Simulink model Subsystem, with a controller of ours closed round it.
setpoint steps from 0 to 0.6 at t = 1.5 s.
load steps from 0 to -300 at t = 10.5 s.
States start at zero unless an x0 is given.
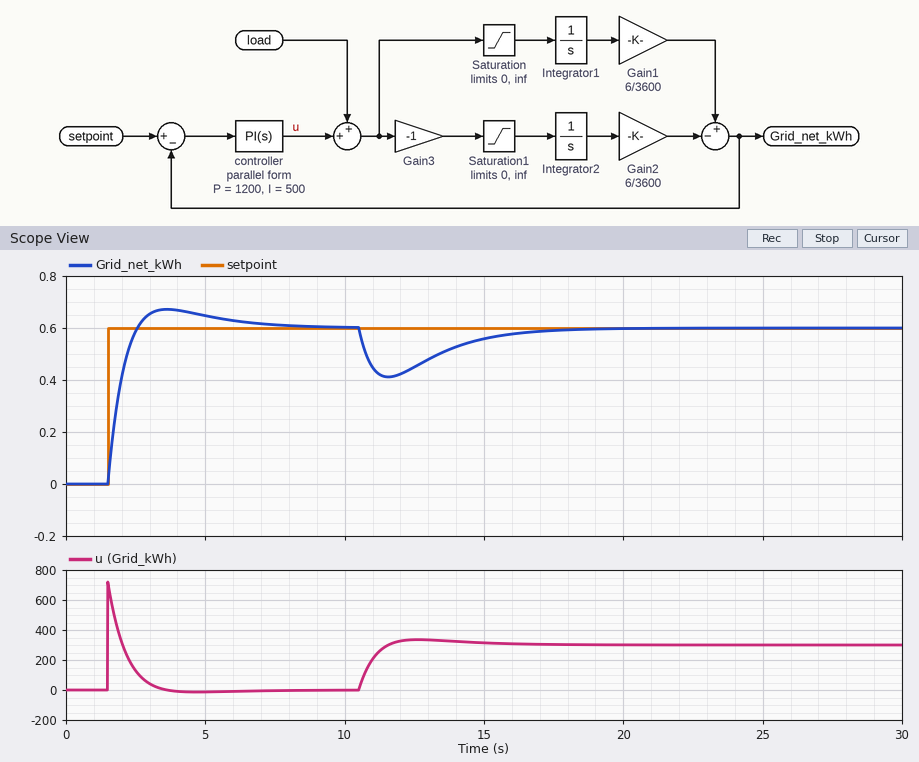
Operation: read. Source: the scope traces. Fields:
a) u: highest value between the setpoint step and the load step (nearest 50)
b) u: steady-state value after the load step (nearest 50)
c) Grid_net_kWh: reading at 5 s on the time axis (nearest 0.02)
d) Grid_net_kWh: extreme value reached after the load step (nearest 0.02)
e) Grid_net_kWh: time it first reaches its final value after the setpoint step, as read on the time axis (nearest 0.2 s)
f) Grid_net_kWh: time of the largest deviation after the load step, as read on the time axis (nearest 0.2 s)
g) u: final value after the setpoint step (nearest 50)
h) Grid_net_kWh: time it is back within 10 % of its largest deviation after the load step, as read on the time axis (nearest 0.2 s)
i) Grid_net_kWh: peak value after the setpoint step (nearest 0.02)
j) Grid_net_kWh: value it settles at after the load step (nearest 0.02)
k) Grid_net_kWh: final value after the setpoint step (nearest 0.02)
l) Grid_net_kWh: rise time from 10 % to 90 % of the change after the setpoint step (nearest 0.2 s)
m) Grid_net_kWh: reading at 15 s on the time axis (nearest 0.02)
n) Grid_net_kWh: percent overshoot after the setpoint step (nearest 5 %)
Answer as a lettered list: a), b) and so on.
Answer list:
a) 700
b) 300
c) 0.64
d) 0.42
e) 2.6 s
f) 11.6 s
g) 0
h) 16.4 s
i) 0.68
j) 0.60
k) 0.60
l) 0.8 s
m) 0.56
n) 10 %
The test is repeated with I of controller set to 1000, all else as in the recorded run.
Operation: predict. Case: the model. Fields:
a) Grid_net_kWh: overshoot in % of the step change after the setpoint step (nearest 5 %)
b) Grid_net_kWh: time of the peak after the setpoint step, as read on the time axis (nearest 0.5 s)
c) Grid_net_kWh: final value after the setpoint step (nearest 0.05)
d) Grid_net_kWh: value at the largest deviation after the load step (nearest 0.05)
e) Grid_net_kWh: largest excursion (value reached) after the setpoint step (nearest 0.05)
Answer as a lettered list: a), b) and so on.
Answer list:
a) 20 %
b) 3.0 s
c) 0.60
d) 0.45
e) 0.70
